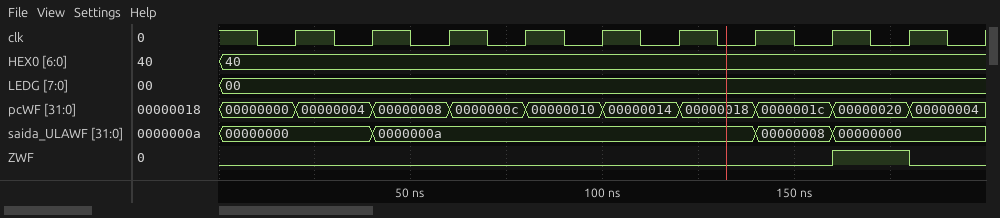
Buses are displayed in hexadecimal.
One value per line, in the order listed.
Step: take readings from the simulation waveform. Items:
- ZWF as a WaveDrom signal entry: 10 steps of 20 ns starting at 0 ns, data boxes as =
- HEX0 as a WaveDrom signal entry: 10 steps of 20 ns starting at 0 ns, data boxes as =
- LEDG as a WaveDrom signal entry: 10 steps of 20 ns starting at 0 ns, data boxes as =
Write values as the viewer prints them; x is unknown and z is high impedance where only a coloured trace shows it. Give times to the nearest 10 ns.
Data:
{name: 'ZWF', wave: '0.......10'}
{name: 'HEX0', wave: '=.........', data: '40'}
{name: 'LEDG', wave: '=.........', data: '00'}
